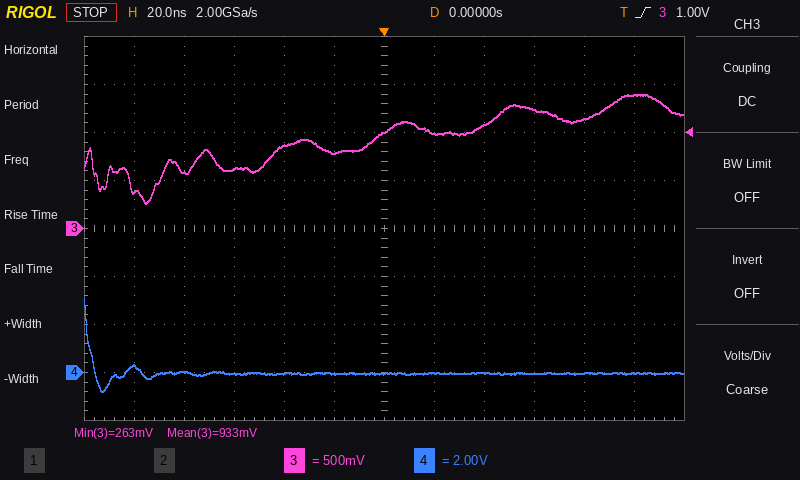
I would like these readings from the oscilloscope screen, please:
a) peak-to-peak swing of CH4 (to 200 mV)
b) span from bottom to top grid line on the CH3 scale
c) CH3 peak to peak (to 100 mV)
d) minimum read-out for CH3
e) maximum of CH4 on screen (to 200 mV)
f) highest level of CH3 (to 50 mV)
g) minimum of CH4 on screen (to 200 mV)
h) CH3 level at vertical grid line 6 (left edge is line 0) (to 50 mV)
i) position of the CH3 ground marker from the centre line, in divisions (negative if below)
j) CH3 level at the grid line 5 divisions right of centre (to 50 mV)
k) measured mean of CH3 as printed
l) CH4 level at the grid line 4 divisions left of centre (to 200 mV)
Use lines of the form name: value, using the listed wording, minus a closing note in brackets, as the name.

peak-to-peak swing of CH4: 3.8 V
span from bottom to top grid line on the CH3 scale: 4 V
CH3 peak to peak: 1.10 V
minimum read-out for CH3: 263 mV
maximum of CH4 on screen: 3.0 V
highest level of CH3: 1.40 V
minimum of CH4 on screen: -800 mV
CH3 level at vertical grid line 6 (left edge is line 0): 1.00 V
position of the CH3 ground marker from the centre line, in divisions: 0.0 div
CH3 level at the grid line 5 divisions right of centre: 1.40 V
measured mean of CH3 as printed: 933 mV
CH4 level at the grid line 4 divisions left of centre: 0.0 V
